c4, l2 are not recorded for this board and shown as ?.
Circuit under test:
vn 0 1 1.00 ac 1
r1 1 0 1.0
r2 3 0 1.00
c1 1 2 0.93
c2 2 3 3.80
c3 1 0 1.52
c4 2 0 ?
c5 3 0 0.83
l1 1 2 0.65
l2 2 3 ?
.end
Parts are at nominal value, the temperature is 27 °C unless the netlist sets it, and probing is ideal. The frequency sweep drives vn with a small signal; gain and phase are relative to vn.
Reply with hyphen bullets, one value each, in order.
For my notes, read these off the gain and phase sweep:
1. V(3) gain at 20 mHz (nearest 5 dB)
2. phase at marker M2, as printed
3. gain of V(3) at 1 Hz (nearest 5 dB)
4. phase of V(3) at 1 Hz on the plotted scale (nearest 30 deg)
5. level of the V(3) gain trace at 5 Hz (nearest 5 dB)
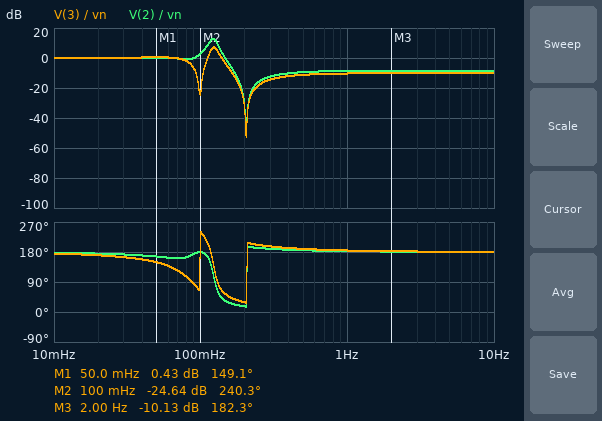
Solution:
- 0 dB
- 240.3 deg
- -10 dB
- 180 deg
- -10 dB
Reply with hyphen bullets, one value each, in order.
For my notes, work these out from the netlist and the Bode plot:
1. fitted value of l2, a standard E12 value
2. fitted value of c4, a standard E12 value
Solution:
- 680 mH
- 820 mF
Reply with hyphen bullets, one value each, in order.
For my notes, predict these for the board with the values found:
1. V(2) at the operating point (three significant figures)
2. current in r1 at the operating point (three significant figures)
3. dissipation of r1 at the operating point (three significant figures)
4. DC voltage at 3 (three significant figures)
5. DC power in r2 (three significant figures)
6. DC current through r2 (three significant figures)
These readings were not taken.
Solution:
- -1.00 V
- 1.00 A
- 1.00 W
- -1.00 V
- 1.00 W
- 1.00 A
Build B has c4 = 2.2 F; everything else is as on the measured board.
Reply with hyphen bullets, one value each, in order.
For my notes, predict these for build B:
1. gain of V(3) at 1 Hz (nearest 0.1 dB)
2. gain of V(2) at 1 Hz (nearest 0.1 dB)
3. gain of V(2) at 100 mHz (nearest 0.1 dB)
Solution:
- -14.3 dB
- -12.5 dB
- 12.6 dB
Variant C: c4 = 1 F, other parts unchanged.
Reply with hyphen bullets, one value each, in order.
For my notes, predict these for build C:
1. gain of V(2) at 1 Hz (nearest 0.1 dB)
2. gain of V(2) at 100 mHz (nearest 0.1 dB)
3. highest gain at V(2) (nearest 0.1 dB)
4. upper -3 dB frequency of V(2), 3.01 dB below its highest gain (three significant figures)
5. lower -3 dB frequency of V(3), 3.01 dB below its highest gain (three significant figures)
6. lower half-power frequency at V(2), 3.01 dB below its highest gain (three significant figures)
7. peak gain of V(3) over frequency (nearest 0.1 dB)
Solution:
- -9.2 dB
- 3.9 dB
- 14.6 dB
- 125 mHz
- 115 mHz
- 113 mHz
- 8.4 dB
